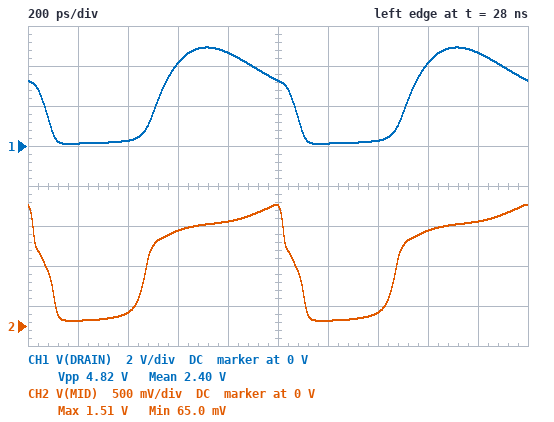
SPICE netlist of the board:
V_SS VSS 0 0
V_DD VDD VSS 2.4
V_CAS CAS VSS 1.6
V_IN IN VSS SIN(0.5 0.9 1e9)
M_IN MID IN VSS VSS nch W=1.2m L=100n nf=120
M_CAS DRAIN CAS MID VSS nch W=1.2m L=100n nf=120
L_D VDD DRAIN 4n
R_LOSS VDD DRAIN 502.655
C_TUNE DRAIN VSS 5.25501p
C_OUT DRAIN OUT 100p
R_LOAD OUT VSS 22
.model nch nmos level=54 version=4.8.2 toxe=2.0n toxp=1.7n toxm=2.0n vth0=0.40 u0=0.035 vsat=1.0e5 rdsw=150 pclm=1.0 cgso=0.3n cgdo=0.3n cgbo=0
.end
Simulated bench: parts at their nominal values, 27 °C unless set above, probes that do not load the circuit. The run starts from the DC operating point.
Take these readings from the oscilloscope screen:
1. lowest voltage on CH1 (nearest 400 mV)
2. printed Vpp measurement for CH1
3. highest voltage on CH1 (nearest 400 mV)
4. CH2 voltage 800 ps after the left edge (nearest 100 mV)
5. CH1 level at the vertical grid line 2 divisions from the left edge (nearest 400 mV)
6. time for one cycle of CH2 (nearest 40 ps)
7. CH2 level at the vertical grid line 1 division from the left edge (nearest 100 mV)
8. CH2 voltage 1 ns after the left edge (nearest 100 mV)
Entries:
0 V
4.82 V
4.8 V
1.3 V
400 mV
1.00 ns
100 mV
1.5 V
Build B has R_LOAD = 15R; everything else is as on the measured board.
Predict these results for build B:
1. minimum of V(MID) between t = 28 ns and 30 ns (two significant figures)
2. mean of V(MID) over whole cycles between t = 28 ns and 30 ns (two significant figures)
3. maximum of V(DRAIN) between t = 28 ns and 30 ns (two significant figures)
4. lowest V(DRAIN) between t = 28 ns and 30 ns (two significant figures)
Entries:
100 mV
840 mV
4.5 V
190 mV
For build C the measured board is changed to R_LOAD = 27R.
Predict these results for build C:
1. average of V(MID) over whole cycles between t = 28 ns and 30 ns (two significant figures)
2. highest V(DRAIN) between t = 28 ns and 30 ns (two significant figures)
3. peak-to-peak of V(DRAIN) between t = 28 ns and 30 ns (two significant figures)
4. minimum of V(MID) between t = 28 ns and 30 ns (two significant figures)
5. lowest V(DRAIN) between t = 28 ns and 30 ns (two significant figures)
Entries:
810 mV
5.1 V
5.0 V
50 mV
86 mV
